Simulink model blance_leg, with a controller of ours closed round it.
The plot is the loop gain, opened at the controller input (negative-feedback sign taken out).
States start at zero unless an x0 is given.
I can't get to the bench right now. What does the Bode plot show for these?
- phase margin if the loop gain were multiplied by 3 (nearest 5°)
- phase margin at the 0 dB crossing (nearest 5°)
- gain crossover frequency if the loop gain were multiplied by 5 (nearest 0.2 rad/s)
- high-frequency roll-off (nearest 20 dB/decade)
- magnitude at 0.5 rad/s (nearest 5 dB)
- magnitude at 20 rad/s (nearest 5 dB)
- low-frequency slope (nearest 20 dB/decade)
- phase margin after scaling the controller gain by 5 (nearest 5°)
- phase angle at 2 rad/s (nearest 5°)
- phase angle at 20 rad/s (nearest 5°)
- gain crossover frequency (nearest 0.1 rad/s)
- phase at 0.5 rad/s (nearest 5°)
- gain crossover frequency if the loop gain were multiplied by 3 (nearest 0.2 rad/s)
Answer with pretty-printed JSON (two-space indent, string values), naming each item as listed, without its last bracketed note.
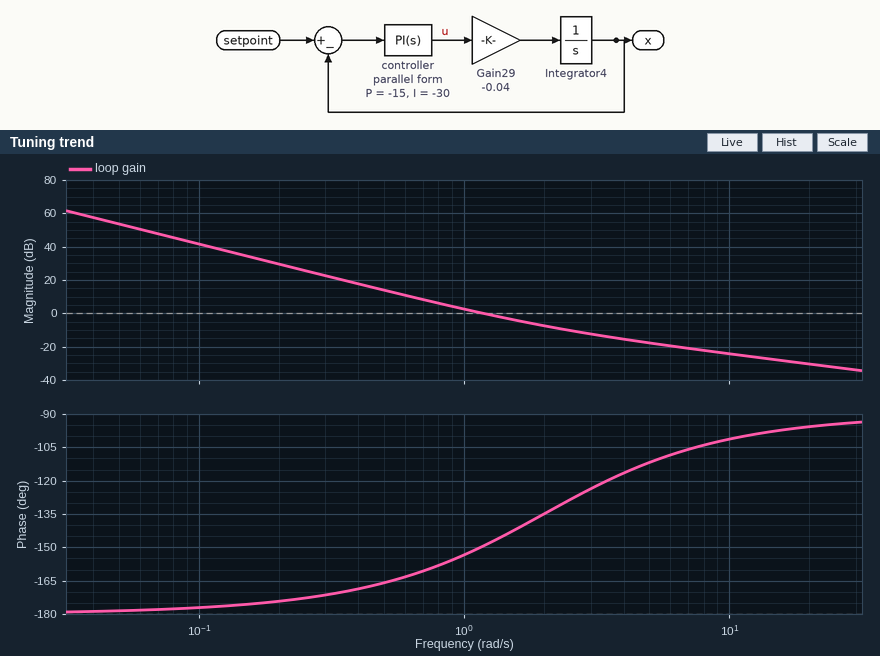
{
  "phase margin if the loop gain were multiplied by 3": "50°",
  "phase margin at the 0 dB crossing": "30°",
  "gain crossover frequency if the loop gain were multiplied by 5": "3.4 rad/s",
  "high-frequency roll-off": "-20 dB/decade",
  "magnitude at 0.5 rad/s": "15 dB",
  "magnitude at 20 rad/s": "-30 dB",
  "low-frequency slope": "-40 dB/decade",
  "phase margin after scaling the controller gain by 5": "60°",
  "phase angle at 2 rad/s": "-135°",
  "phase angle at 20 rad/s": "-95°",
  "gain crossover frequency": "1.2 rad/s",
  "phase at 0.5 rad/s": "-165°",
  "gain crossover frequency if the loop gain were multiplied by 3": "2.4 rad/s"
}
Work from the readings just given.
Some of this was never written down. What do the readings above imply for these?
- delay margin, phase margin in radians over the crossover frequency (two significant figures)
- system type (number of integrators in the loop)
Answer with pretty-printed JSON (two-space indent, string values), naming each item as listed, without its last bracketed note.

{
  "delay margin, phase margin in radians over the crossover frequency": "0.44 s",
  "system type": "2"
}
